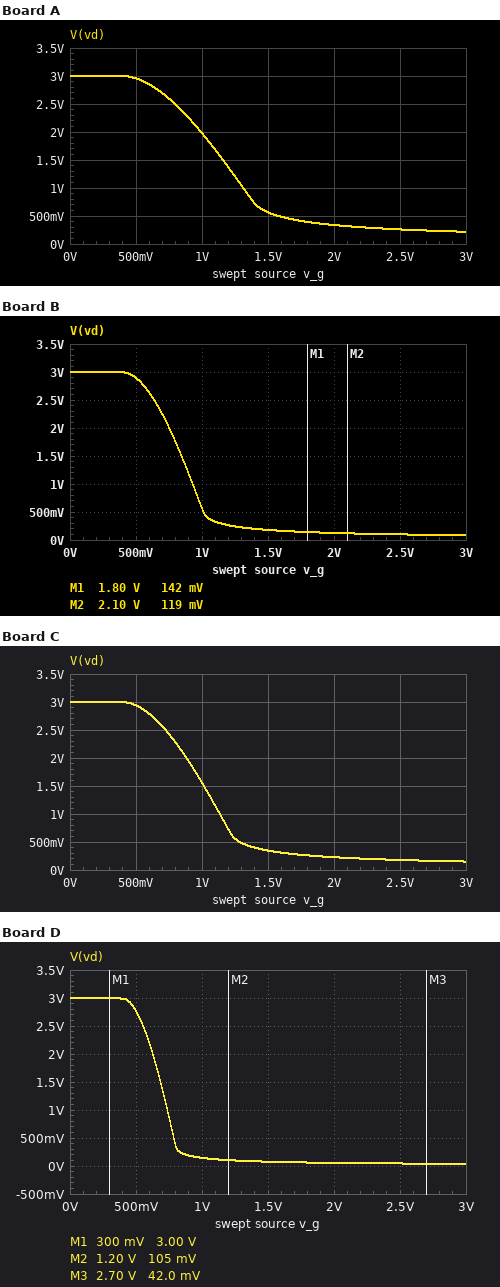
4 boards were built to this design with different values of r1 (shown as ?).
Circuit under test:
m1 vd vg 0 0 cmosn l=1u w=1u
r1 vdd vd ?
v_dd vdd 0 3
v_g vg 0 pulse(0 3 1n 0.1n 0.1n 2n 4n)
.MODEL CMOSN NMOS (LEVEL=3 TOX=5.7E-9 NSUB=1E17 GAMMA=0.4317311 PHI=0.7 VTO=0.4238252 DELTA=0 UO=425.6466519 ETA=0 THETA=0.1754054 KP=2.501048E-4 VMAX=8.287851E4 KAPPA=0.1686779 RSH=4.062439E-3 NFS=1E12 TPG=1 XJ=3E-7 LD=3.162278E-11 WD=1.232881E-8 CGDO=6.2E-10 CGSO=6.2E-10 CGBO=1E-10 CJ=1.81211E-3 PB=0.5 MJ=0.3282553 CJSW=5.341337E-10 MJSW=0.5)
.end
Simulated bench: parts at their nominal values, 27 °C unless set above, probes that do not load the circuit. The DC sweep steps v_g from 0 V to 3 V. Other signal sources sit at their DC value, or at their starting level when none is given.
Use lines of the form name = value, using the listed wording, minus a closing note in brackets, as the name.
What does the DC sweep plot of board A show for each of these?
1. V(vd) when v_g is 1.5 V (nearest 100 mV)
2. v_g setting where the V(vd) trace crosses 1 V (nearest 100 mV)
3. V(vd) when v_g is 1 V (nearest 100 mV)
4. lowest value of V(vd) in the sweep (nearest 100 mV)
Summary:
V(vd) when v_g is 1.5 V = 600 mV
v_g setting where the V(vd) trace crosses 1 V = 1.3 V
V(vd) when v_g is 1 V = 2.0 V
lowest value of V(vd) in the sweep = 200 mV
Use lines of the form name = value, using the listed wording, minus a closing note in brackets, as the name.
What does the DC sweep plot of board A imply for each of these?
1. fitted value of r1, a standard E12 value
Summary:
fitted value of r1, a standard E12 value = 33 kΩ
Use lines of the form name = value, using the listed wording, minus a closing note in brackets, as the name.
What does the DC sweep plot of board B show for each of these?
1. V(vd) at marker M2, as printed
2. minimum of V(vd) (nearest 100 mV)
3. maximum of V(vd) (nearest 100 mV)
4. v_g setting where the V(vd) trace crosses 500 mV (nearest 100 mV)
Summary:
V(vd) at marker M2, as printed = 119 mV
minimum of V(vd) = 100 mV
maximum of V(vd) = 3.0 V
v_g setting where the V(vd) trace crosses 500 mV = 1.0 V
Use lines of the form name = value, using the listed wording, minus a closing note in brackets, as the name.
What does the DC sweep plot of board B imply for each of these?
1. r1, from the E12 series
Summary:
r1, from the E12 series = 82 kΩ
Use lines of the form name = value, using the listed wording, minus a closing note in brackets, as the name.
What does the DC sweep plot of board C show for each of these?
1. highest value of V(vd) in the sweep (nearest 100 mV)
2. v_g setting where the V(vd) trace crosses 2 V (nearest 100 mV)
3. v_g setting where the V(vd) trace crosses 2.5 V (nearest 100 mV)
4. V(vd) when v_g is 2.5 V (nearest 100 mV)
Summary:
highest value of V(vd) in the sweep = 3.0 V
v_g setting where the V(vd) trace crosses 2 V = 900 mV
v_g setting where the V(vd) trace crosses 2.5 V = 700 mV
V(vd) when v_g is 2.5 V = 200 mV
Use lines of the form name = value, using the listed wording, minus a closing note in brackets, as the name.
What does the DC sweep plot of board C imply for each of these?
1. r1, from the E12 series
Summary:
r1, from the E12 series = 47 kΩ
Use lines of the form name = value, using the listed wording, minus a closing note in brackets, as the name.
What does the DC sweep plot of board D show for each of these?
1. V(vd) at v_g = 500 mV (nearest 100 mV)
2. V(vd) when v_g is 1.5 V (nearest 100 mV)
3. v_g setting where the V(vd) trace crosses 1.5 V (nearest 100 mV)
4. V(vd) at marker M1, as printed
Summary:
V(vd) at v_g = 500 mV = 2.8 V
V(vd) when v_g is 1.5 V = 100 mV
v_g setting where the V(vd) trace crosses 1.5 V = 700 mV
V(vd) at marker M1, as printed = 3.00 V
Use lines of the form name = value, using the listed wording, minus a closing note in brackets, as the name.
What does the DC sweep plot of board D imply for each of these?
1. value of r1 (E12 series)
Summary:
value of r1 = 180 kΩ
